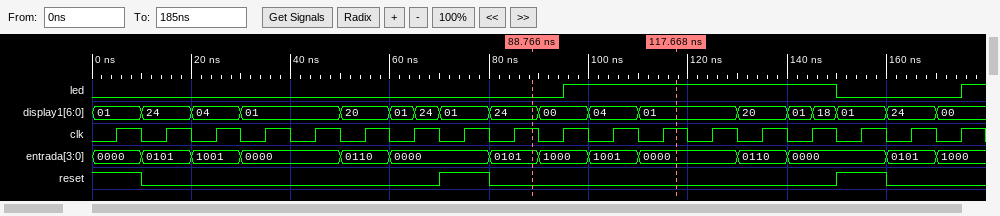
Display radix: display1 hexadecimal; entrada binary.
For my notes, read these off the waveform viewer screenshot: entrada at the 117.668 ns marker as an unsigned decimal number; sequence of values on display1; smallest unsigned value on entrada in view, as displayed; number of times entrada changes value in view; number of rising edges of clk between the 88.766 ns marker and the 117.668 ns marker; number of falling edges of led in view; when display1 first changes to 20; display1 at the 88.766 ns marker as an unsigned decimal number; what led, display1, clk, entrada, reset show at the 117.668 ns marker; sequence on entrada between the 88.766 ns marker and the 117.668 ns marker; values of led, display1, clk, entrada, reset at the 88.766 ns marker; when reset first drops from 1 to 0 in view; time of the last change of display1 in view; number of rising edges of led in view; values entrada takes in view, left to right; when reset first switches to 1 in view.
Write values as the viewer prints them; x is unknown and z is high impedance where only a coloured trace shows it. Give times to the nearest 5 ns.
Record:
0
01, 24, 04, 01, 20, 01, 24, 01, 24, 00, 04, 01, 20, 01, 18, 01, 24, 00
0000
13
3
1
50 ns
36
led=1, display1=01, clk=1, entrada=0000, reset=0
0101, 1000, 1001, 0000
led=0, display1=24, clk=1, entrada=0101, reset=0
10 ns
170 ns
2
0000, 0101, 1001, 0000, 0110, 0000, 0101, 1000, 1001, 0000, 0110, 0000, 0101, 1000
70 ns
